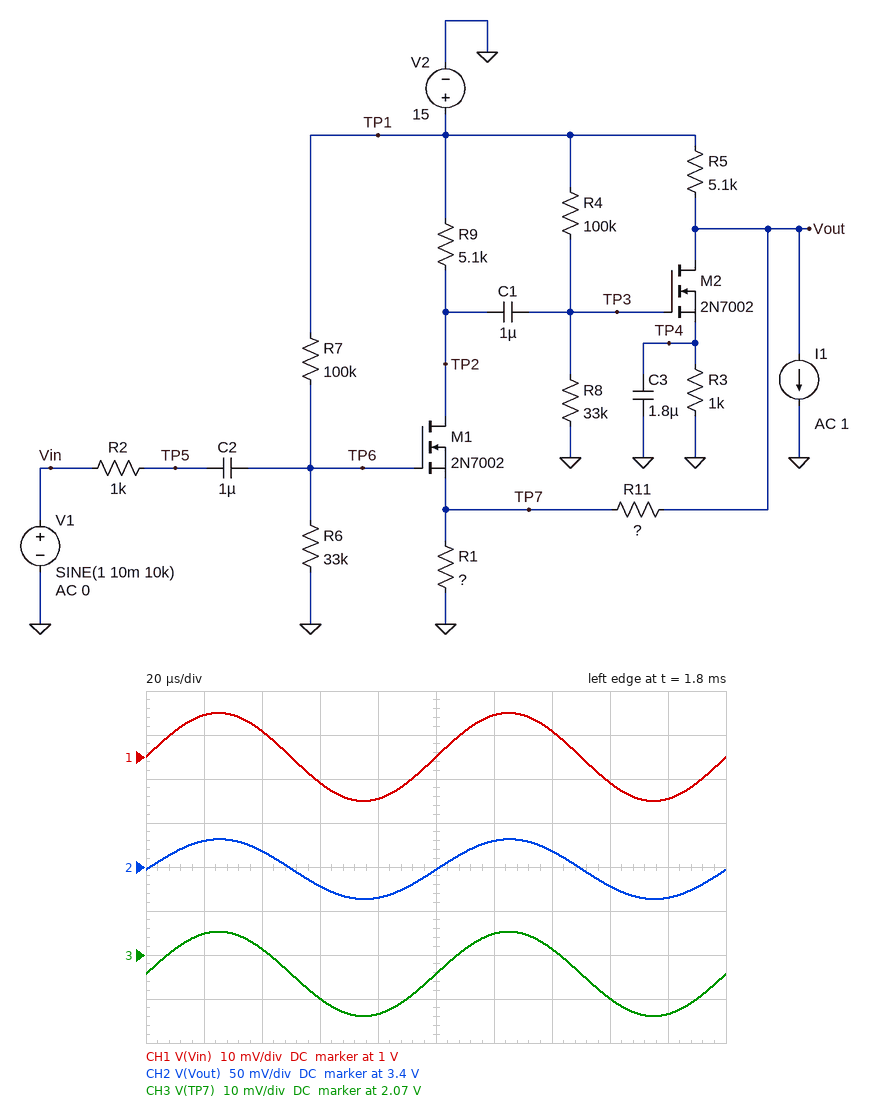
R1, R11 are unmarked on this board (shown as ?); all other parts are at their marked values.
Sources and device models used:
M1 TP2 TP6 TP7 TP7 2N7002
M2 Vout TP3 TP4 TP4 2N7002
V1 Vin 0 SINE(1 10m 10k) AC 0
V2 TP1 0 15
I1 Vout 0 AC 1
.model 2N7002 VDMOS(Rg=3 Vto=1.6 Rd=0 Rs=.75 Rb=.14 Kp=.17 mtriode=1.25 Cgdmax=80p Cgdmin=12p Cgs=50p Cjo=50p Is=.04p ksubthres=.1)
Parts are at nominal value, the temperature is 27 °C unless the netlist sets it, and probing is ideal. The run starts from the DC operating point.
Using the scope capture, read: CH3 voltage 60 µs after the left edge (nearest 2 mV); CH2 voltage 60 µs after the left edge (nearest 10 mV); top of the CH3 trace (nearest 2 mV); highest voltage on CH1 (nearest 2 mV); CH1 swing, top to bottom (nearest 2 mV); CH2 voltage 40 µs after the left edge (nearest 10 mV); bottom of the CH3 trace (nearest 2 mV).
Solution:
2.060 V
3.38 V
2.076 V
1.010 V
20 mV
3.42 V
2.056 V
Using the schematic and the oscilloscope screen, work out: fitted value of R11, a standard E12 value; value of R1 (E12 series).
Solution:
4.7 kΩ
1.8 kΩ
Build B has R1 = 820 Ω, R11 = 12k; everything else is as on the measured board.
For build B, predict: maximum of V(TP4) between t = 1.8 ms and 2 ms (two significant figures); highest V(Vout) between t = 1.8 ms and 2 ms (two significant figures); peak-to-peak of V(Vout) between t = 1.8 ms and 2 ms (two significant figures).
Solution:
2.0 V
4.1 V
290 mV
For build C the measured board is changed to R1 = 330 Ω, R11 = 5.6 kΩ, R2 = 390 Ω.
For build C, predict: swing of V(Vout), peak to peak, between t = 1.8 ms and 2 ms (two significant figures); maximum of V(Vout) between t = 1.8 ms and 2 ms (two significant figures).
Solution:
2.9 mV
3.0 V
